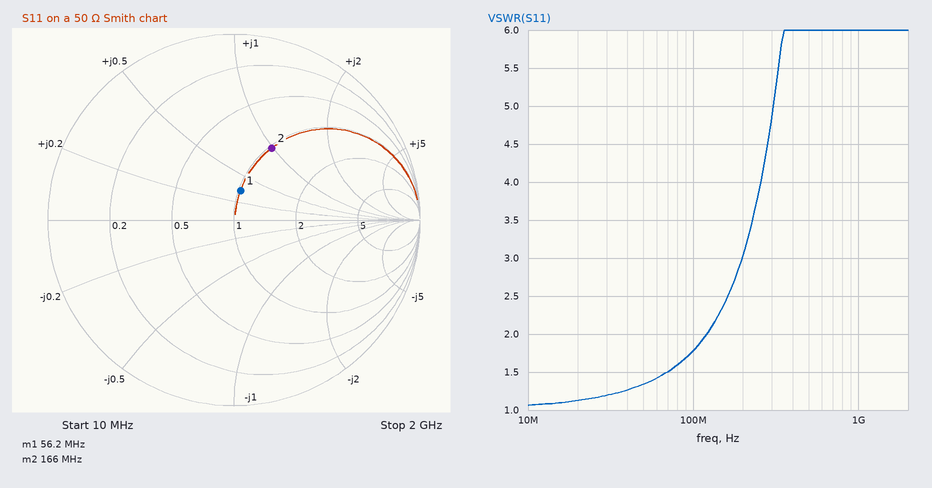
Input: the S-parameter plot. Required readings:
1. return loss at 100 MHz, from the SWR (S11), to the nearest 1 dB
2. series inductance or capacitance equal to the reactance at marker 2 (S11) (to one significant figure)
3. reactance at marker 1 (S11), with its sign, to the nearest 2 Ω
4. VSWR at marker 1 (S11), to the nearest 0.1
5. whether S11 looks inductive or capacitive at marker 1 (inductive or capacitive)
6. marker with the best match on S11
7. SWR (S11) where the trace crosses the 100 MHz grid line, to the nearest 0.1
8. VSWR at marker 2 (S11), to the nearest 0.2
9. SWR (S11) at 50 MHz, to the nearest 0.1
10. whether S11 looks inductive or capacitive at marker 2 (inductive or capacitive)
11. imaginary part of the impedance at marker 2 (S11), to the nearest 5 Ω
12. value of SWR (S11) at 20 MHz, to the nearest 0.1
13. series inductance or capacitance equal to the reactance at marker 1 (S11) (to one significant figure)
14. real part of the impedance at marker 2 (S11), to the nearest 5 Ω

11 dB
50 nH
+16 Ω
1.4
inductive
marker 1
1.8
2.6
1.3
inductive
+50 Ω
1.1
50 nH
50 Ω
